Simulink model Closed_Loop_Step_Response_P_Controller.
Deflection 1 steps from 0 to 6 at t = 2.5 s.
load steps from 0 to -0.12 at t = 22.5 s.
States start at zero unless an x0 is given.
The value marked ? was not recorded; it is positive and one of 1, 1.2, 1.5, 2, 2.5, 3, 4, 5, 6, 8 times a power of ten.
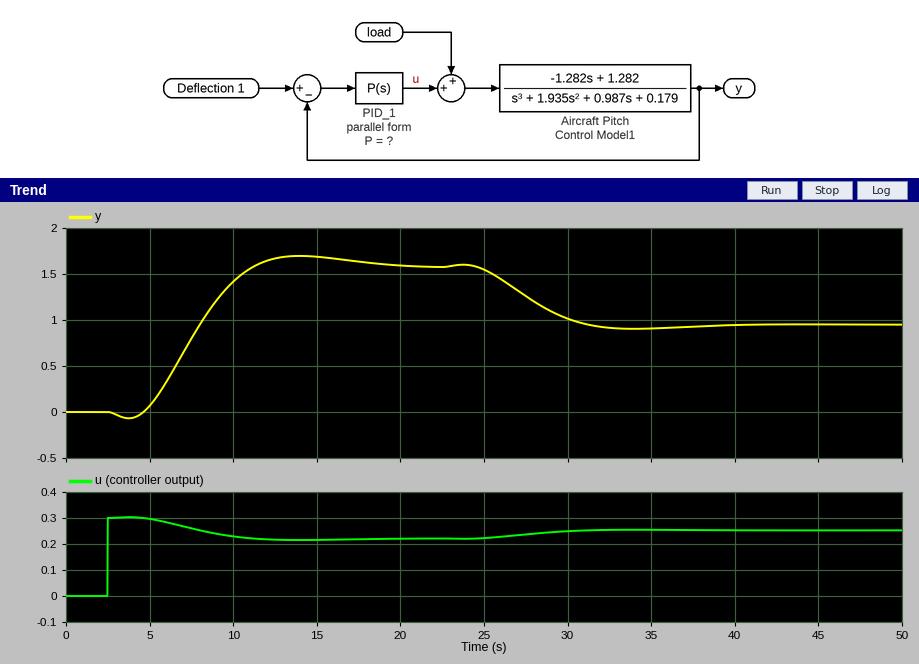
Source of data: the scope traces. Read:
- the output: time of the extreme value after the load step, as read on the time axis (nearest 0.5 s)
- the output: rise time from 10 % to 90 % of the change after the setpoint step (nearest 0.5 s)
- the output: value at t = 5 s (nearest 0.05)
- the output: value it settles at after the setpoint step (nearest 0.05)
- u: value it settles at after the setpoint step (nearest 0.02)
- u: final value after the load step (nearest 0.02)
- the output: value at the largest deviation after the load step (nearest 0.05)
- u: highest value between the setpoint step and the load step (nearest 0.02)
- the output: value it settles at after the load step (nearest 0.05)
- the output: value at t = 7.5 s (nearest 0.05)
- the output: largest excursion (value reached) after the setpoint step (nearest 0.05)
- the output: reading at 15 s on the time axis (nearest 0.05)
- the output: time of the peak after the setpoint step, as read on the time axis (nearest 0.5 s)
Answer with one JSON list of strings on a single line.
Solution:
["34.0 s", "4.5 s", "0.05", "1.60", "0.22", "0.26", "0.90", "0.30", "0.95", "0.80", "1.70", "1.70", "14.0 s"]
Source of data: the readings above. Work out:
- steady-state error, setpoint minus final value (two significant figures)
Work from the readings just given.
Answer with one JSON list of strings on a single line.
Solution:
["4.4"]
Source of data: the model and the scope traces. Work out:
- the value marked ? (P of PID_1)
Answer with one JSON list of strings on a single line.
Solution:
["0.05"]
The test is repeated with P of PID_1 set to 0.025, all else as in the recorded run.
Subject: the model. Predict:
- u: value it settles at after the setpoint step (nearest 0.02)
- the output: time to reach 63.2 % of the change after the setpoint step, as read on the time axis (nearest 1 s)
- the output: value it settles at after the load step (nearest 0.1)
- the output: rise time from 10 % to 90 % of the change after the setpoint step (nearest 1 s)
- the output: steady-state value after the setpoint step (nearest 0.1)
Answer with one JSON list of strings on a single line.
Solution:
["0.12", "9 s", "0.2", "6 s", "0.9"]
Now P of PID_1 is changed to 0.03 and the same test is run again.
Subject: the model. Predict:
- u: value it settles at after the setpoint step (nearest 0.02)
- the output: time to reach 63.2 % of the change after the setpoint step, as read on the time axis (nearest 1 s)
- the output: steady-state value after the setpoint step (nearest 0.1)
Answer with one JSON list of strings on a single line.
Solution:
["0.14", "9 s", "1.1"]
